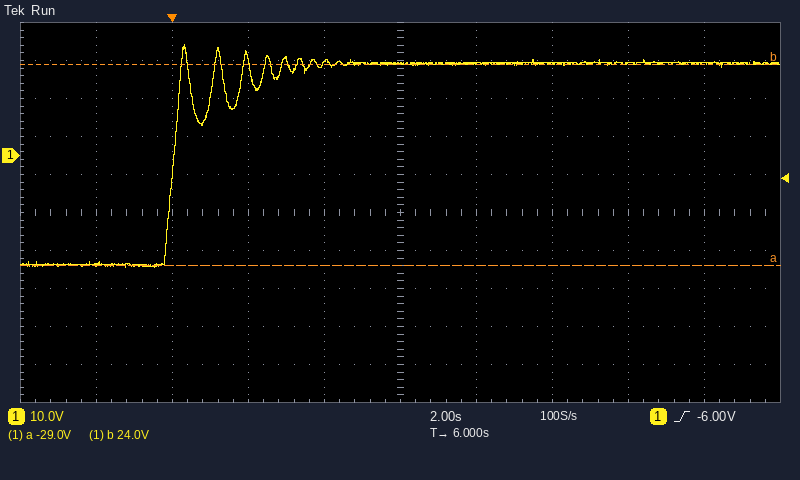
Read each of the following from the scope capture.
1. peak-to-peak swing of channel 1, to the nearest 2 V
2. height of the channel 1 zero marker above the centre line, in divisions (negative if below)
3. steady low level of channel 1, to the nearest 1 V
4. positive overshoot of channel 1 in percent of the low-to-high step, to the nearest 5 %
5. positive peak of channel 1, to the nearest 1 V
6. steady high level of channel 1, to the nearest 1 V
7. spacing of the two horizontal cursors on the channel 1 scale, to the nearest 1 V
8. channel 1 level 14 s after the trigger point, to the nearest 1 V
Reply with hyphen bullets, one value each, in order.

- 58 V
- +1.5 div
- -29 V
- 10 %
- 29 V
- 24 V
- 53 V
- 24 V
